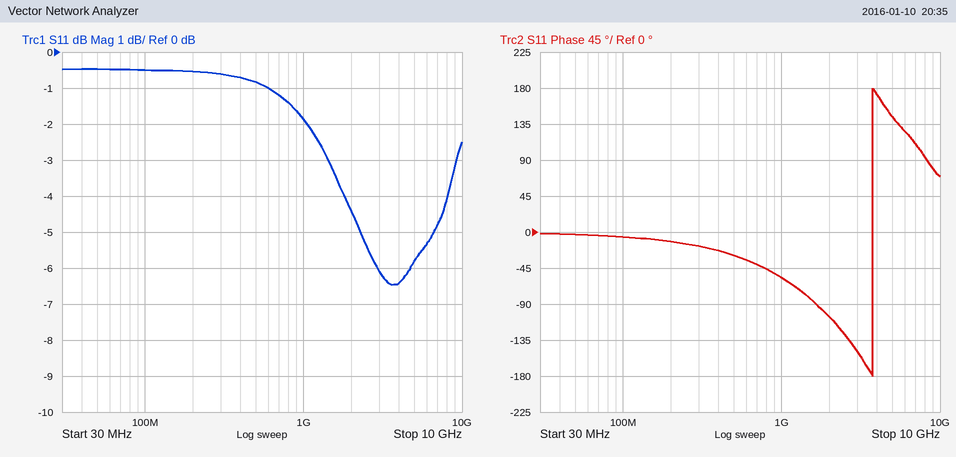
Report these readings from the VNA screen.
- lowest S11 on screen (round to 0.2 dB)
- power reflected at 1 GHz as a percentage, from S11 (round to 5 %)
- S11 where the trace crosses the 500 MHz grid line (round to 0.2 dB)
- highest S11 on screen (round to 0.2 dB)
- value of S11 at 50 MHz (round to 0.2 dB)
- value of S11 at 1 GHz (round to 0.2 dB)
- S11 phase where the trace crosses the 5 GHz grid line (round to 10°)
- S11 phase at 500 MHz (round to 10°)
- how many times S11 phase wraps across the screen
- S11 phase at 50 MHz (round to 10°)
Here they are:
-6.4 dB
65 %
-0.8 dB
-0.4 dB
-0.4 dB
-1.8 dB
140°
-30°
1
0°
